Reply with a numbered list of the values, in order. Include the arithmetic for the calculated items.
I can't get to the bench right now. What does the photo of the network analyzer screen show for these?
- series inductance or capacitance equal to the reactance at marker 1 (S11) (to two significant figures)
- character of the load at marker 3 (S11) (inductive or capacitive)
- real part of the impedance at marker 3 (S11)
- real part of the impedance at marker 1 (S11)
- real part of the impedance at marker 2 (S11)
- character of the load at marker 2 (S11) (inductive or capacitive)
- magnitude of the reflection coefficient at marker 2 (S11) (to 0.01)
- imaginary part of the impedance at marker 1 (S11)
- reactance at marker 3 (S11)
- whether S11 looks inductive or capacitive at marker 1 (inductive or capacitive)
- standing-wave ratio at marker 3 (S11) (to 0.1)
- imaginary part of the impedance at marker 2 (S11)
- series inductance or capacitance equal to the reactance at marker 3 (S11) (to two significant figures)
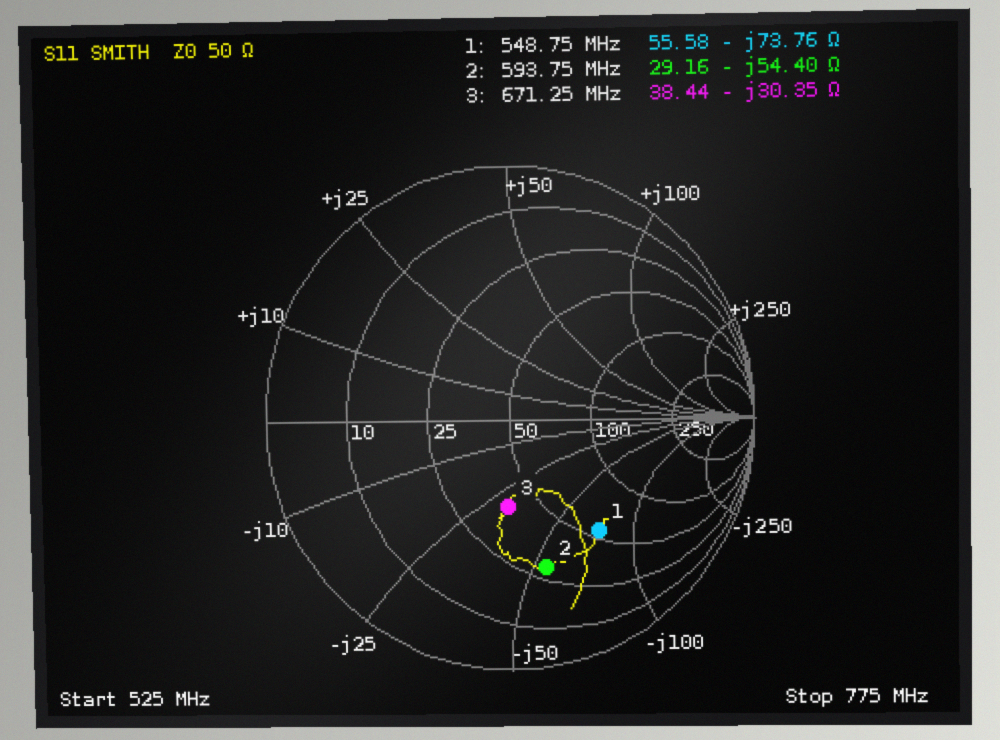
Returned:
1. C = 1/(2π × 548.75 MHz × 73.76 Ω) ≈ 3.9 pF
2. capacitive
3. 38.44 Ω
4. 55.58 Ω
5. 29.16 Ω
6. capacitive
7. 0.61
8. -73.76 Ω
9. -30.35 Ω
10. capacitive
11. 2.1
12. -54.40 Ω
13. C = 1/(2π × 671.25 MHz × 30.35 Ω) ≈ 7.8 pF
